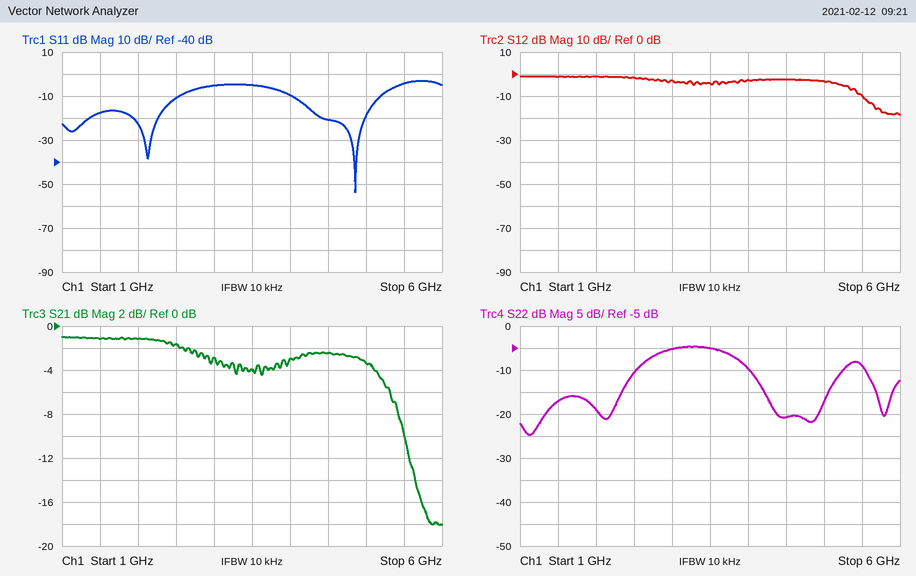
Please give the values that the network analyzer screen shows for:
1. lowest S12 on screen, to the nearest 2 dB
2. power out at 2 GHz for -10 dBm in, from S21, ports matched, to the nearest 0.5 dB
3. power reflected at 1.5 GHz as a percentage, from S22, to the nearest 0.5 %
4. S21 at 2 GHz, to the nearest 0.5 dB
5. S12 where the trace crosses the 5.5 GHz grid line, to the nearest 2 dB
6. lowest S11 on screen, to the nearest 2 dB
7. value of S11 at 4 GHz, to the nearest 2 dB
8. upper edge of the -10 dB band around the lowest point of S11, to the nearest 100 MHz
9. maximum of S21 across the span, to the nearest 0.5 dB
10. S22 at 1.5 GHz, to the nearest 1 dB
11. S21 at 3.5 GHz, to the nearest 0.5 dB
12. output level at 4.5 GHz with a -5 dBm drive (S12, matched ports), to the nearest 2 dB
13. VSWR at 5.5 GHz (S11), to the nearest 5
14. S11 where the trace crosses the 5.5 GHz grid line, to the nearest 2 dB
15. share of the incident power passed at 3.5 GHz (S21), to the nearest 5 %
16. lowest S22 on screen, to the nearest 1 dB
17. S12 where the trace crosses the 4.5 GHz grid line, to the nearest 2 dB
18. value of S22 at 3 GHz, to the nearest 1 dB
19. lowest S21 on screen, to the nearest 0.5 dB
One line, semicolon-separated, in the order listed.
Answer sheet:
-18 dB; -11.0 dBm; 2.0 %; -1.0 dB; -10 dB; -54 dB; -10 dB; 5.2 GHz; -1.0 dB; -17 dB; -4.0 dB; -8 dBm; 5; -4 dB; 40 %; -25 dB; -2 dB; -5 dB; -18.0 dB
